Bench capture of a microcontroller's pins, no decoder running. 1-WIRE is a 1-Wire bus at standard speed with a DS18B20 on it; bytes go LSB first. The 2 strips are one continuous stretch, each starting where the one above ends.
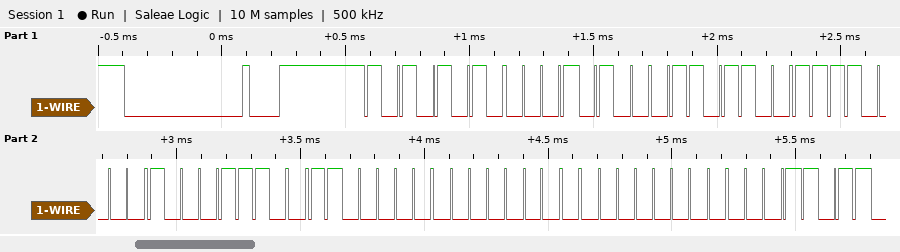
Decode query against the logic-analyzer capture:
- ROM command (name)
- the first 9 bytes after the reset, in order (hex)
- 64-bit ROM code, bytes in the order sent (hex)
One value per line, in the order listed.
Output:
Match ROM
55 28 36 0F 71 06 00 00 D8
28 36 0F 71 06 00 00 D8
